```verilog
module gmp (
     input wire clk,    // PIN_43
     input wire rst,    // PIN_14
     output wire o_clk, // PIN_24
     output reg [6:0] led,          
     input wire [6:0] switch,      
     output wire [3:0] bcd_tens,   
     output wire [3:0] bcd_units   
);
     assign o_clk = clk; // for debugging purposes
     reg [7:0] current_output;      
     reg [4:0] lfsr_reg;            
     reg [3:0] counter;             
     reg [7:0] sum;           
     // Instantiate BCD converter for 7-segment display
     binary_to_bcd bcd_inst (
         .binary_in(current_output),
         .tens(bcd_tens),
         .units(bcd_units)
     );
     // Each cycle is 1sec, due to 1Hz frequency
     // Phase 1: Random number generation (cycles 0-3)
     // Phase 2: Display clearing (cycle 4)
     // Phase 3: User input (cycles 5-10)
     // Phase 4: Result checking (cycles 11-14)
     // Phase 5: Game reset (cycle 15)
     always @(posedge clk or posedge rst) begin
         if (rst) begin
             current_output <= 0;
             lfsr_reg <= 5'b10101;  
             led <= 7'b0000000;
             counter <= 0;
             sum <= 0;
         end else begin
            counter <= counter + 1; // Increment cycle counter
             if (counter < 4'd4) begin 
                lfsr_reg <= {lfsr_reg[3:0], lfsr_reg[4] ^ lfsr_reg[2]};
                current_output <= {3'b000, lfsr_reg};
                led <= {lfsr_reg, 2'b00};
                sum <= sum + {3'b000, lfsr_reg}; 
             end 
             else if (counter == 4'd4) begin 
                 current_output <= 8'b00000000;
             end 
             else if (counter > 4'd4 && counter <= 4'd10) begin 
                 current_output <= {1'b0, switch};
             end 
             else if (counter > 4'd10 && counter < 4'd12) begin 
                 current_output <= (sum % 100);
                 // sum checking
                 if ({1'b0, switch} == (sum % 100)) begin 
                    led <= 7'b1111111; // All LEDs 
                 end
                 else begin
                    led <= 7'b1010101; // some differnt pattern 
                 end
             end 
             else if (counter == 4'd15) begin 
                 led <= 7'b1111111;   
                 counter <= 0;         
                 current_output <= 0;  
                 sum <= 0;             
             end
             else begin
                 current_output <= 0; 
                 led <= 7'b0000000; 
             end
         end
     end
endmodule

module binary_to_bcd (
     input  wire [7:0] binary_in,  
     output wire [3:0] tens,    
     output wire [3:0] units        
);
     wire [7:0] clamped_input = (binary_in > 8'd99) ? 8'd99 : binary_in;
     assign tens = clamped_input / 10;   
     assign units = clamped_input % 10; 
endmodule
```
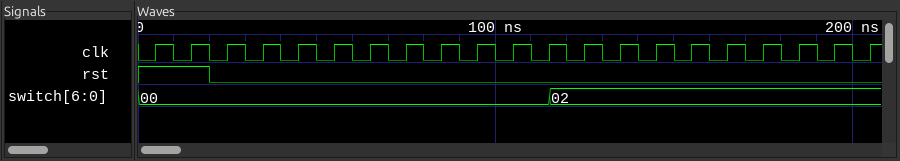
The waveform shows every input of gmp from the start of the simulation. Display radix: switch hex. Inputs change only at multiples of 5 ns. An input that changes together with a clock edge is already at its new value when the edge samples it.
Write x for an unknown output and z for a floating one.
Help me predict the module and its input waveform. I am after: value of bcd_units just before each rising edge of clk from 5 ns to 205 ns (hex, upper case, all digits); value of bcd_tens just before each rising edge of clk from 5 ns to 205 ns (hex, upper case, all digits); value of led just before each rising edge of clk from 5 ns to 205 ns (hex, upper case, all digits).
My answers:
0, 0, 0, 1, 0, 0, 8, 0, 0, 0, 0, 0, 2, 2, 9, 0, 0, 0, 0, 6, 1
0, 0, 0, 2, 1, 2, 0, 0, 0, 0, 0, 0, 0, 0, 5, 0, 0, 0, 0, 1, 0
00, 00, 00, 54, 28, 50, 20, 20, 20, 20, 20, 20, 20, 20, 55, 00, 00, 00, 7F, 40, 04
